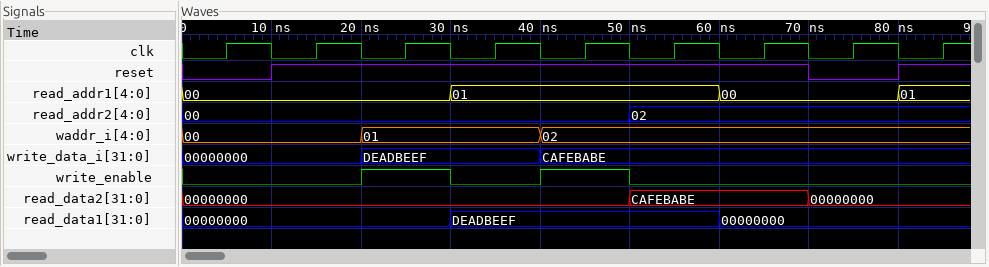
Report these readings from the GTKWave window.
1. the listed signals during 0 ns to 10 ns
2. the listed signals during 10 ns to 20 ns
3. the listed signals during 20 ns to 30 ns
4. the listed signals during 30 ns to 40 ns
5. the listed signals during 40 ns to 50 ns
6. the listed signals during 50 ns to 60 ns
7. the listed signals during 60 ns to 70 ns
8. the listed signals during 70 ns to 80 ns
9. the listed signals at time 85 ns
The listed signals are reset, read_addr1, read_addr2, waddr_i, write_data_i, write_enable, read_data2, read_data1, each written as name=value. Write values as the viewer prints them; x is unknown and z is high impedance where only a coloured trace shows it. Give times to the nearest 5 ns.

reset=0, read_addr1=00, read_addr2=00, waddr_i=00, write_data_i=00000000, write_enable=0, read_data2=00000000, read_data1=00000000
reset=1, read_addr1=00, read_addr2=00, waddr_i=00, write_data_i=00000000, write_enable=0, read_data2=00000000, read_data1=00000000
reset=1, read_addr1=00, read_addr2=00, waddr_i=01, write_data_i=DEADBEEF, write_enable=1, read_data2=00000000, read_data1=00000000
reset=1, read_addr1=01, read_addr2=00, waddr_i=01, write_data_i=DEADBEEF, write_enable=0, read_data2=00000000, read_data1=DEADBEEF
reset=1, read_addr1=01, read_addr2=00, waddr_i=02, write_data_i=CAFEBABE, write_enable=1, read_data2=00000000, read_data1=DEADBEEF
reset=1, read_addr1=01, read_addr2=02, waddr_i=02, write_data_i=CAFEBABE, write_enable=0, read_data2=CAFEBABE, read_data1=DEADBEEF
reset=1, read_addr1=00, read_addr2=02, waddr_i=02, write_data_i=CAFEBABE, write_enable=0, read_data2=CAFEBABE, read_data1=00000000
reset=0, read_addr1=00, read_addr2=02, waddr_i=02, write_data_i=CAFEBABE, write_enable=0, read_data2=00000000, read_data1=00000000
reset=1, read_addr1=01, read_addr2=02, waddr_i=02, write_data_i=CAFEBABE, write_enable=0, read_data2=00000000, read_data1=00000000
